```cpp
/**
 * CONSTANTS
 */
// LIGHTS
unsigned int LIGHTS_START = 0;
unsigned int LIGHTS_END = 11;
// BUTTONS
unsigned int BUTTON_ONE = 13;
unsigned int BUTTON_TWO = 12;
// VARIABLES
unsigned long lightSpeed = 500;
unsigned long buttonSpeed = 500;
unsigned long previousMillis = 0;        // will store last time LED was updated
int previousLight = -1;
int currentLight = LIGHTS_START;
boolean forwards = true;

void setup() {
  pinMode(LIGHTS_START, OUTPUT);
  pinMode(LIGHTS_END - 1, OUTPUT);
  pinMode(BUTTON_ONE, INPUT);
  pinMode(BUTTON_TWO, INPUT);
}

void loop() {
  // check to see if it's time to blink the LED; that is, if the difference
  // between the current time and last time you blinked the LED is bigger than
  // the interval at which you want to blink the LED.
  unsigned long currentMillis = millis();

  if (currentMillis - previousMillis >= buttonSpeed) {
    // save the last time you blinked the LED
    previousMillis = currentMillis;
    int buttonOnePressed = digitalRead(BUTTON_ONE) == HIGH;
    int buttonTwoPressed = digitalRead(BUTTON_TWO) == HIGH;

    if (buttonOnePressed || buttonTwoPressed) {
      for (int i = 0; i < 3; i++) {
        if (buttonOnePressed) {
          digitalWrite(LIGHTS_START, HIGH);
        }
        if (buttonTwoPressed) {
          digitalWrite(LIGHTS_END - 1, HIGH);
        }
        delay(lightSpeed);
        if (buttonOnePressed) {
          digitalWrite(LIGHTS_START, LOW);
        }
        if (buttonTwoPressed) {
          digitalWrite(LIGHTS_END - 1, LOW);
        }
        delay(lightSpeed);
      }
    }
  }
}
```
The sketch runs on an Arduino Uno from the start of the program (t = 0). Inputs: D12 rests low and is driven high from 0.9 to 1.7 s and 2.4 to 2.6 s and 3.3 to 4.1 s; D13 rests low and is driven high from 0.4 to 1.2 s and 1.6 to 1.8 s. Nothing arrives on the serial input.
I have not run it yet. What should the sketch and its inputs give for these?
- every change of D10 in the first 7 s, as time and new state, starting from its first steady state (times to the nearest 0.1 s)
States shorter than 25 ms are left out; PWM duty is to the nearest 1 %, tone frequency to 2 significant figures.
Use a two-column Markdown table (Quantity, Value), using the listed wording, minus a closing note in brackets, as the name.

| Quantity | Value |
|---|---|
| every change of D10 in the first 7 s, as time and new state, starting from its first steady state | 0 s low; 3.5 s high; 4 s low; 4.5 s high; 5 s low; 5.5 s high; 6 s low |
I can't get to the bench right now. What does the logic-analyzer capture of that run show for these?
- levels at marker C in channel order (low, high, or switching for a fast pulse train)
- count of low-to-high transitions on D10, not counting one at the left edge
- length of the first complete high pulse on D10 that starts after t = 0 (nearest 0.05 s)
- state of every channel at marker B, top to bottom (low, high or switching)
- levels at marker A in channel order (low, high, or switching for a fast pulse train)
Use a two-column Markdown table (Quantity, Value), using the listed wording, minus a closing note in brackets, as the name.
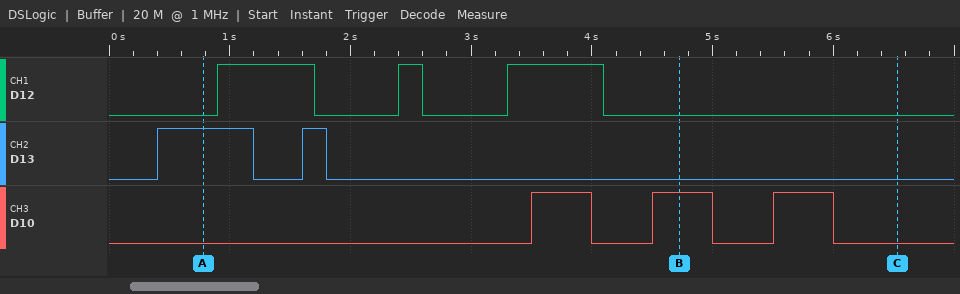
| Quantity | Value |
|---|---|
| levels at marker C in channel order | D12 low, D13 low, D10 low |
| count of low-to-high transitions on D10, not counting one at the left edge | 3 |
| length of the first complete high pulse on D10 that starts after t = 0 | 0.50 s |
| state of every channel at marker B, top to bottom | D12 low, D13 low, D10 high |
| levels at marker A in channel order | D12 low, D13 high, D10 low |
